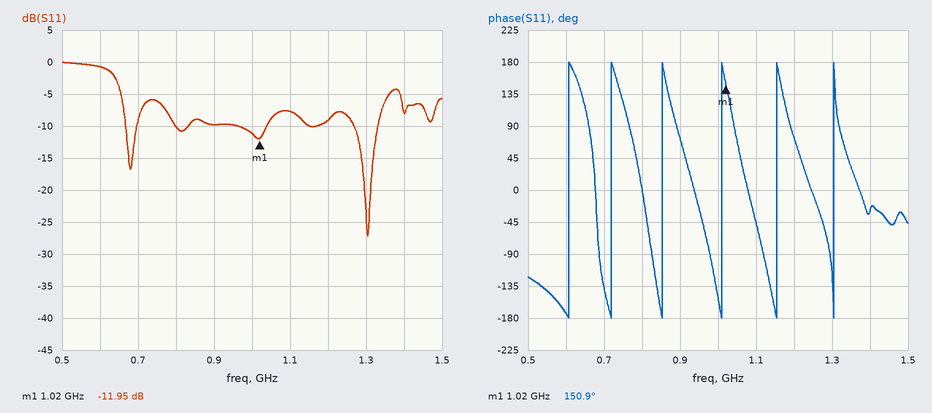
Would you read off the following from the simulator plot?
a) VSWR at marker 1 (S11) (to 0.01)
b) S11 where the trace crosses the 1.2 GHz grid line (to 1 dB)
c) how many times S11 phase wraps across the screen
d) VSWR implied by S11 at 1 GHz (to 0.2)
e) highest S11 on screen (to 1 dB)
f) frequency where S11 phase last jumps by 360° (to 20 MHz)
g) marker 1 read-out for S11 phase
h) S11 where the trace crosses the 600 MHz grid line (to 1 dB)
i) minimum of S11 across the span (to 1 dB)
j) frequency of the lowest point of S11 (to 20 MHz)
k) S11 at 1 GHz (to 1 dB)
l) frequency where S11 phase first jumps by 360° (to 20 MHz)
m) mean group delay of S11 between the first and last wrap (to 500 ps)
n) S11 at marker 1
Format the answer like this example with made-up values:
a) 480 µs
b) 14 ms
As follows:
a) 1.68
b) -9 dB
c) 6
d) 1.8
e) 0 dB
f) 1.30 GHz
g) 150.9°
h) -1 dB
i) -27 dB
j) 1.30 GHz
k) -11 dB
l) 600 MHz
m) 7.0 ns
n) -11.95 dB
